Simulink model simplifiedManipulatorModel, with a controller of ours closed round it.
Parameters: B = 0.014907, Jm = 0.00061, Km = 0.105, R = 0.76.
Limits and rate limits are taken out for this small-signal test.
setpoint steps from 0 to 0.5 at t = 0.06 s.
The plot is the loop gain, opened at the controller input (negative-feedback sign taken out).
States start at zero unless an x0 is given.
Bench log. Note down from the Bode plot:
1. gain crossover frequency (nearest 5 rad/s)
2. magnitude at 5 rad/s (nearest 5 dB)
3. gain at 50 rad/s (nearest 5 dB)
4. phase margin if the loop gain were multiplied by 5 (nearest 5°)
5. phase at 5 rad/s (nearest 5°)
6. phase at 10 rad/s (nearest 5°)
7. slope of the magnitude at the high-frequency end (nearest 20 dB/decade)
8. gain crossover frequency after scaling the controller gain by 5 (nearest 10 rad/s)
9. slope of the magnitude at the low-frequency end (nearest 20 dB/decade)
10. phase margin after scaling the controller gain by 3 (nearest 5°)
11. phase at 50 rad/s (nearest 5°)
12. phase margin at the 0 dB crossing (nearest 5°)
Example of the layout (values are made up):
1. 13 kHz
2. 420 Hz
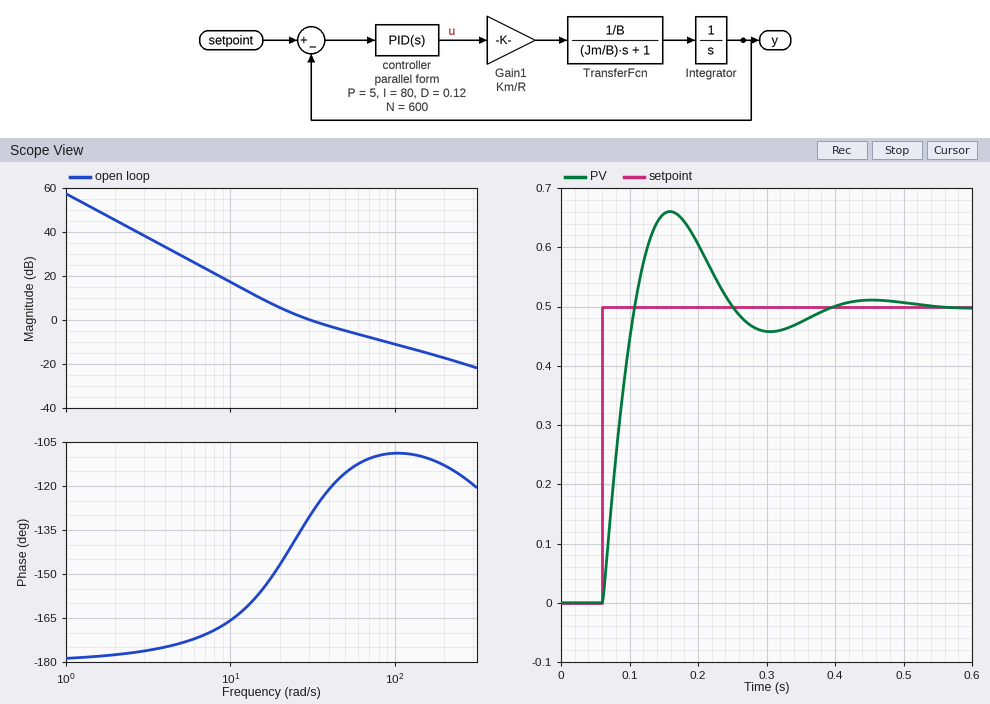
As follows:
1. 30 rad/s
2. 30 dB
3. -5 dB
4. 70°
5. -175°
6. -165°
7. -20 dB/decade
8. 140 rad/s
9. -40 dB/decade
10. 70°
11. -115°
12. 50°
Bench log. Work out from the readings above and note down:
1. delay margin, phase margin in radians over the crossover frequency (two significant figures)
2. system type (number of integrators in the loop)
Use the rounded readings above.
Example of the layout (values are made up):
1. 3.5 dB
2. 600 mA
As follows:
1. 0.029 s
2. 2
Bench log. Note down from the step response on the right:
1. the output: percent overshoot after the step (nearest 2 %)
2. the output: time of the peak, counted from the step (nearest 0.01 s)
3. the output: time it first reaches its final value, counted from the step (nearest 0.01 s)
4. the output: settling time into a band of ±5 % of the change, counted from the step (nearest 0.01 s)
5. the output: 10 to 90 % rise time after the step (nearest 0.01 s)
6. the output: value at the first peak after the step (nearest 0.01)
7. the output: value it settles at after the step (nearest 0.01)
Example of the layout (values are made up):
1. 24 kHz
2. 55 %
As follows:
1. 32 %
2. 0.10 s
3. 0.05 s
4. 0.29 s
5. 0.04 s
6. 0.66
7. 0.50
